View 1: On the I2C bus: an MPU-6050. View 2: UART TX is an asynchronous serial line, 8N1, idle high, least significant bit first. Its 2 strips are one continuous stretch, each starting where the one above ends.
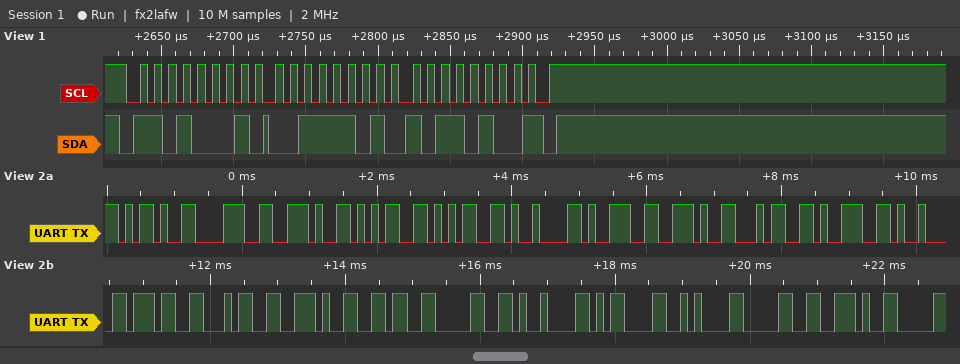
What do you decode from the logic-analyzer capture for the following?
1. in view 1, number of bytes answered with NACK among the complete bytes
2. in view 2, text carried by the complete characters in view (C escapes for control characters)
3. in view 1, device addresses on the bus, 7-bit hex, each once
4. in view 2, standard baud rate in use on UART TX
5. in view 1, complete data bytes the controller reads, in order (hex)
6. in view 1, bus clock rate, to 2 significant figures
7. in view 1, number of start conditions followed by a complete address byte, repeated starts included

1
"-8.55\t9.49\t74.60\t\r\n0."
0x68
9600 baud
3D B4
100 kHz
1
